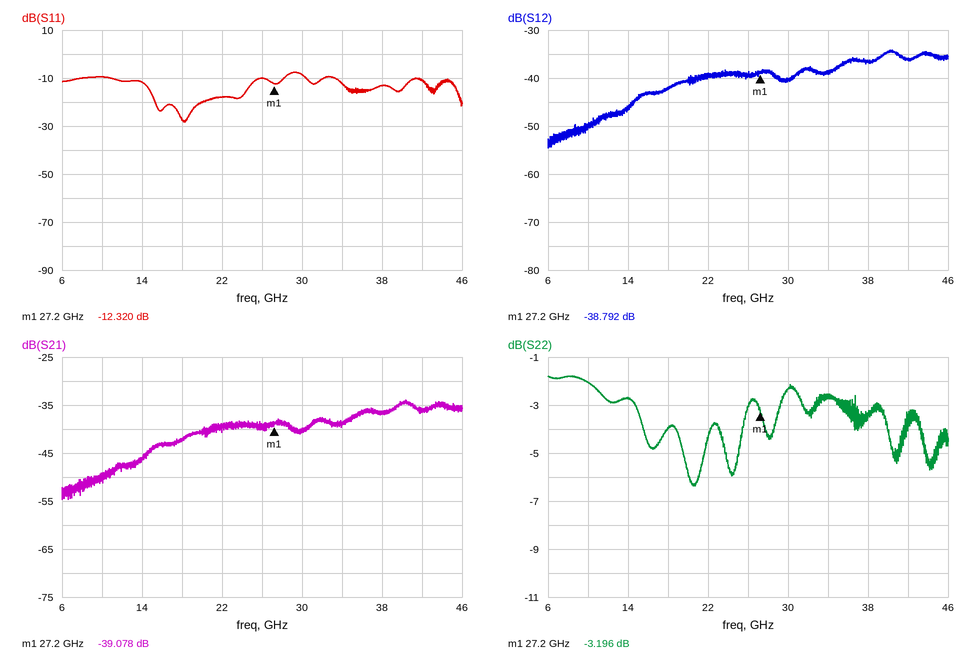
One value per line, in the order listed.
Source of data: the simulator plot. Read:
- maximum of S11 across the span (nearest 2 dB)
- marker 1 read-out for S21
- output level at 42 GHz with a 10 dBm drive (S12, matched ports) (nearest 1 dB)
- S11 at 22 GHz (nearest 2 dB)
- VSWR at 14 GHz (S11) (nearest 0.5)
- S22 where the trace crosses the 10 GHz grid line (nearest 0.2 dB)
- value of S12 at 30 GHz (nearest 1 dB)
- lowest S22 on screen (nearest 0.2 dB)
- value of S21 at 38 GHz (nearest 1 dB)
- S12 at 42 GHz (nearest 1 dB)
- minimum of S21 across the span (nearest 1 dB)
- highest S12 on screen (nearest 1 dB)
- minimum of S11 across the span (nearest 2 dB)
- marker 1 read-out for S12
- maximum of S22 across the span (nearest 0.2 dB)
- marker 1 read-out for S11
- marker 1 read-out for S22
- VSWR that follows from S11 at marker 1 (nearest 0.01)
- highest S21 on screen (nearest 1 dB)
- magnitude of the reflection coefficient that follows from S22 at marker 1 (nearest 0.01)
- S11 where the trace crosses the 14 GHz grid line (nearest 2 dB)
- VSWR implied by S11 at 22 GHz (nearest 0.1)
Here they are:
-8 dB
-39.078 dB
-26 dBm
-18 dB
1.5
-2.0 dB
-40 dB
-6.4 dB
-37 dB
-36 dB
-55 dB
-34 dB
-28 dB
-38.792 dB
-1.8 dB
-12.320 dB
-3.196 dB
1.64
-34 dB
0.69
-12 dB
1.3
